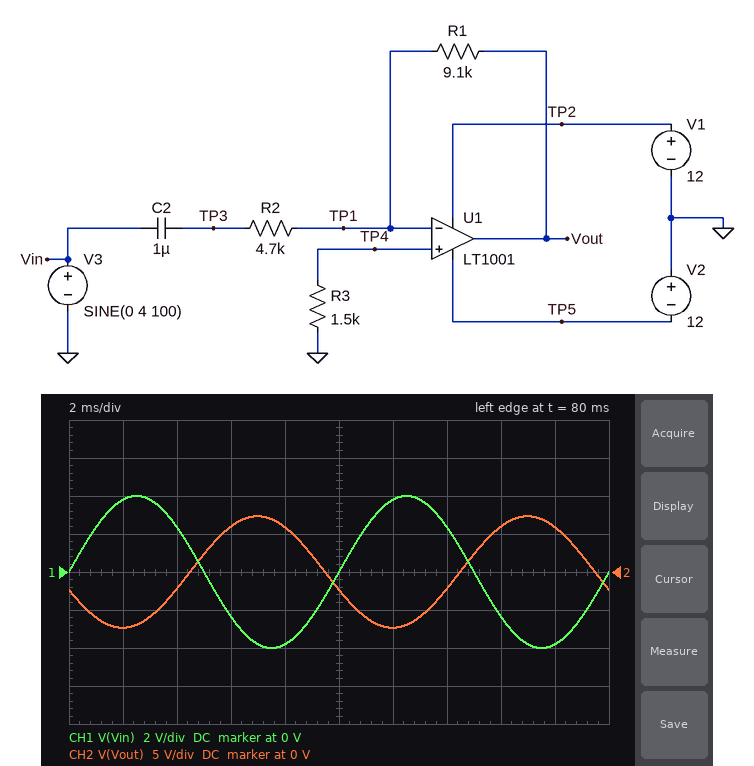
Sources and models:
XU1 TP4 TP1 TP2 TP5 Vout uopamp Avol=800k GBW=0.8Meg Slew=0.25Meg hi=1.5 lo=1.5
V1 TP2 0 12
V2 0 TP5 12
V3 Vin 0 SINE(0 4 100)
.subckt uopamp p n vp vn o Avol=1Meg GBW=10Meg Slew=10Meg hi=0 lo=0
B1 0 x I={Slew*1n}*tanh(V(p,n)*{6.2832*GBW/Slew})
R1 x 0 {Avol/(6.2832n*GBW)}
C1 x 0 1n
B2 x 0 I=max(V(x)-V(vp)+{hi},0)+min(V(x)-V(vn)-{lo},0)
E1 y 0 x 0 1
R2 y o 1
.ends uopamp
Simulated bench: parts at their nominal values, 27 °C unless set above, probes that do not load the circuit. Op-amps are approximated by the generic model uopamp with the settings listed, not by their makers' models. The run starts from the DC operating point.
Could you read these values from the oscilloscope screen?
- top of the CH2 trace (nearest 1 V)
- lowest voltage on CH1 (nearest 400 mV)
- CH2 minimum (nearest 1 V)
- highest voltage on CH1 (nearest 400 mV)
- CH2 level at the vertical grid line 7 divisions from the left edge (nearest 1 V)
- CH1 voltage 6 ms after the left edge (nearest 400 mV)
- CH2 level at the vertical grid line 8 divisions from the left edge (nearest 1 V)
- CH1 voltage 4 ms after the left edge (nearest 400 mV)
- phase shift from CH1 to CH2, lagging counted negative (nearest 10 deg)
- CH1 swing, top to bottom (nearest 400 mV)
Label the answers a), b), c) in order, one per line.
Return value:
a) 7 V
b) -4.0 V
c) -7 V
d) 4.0 V
e) -2 V
f) -2.4 V
g) 6 V
h) 2.4 V
i) -160 deg
j) 8.0 V
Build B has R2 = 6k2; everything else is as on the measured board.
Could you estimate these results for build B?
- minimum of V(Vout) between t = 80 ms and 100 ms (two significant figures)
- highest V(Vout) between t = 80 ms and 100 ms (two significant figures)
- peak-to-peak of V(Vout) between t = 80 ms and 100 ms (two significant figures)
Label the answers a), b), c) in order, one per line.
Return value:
a) -5.7 V
b) 5.7 V
c) 11 V
